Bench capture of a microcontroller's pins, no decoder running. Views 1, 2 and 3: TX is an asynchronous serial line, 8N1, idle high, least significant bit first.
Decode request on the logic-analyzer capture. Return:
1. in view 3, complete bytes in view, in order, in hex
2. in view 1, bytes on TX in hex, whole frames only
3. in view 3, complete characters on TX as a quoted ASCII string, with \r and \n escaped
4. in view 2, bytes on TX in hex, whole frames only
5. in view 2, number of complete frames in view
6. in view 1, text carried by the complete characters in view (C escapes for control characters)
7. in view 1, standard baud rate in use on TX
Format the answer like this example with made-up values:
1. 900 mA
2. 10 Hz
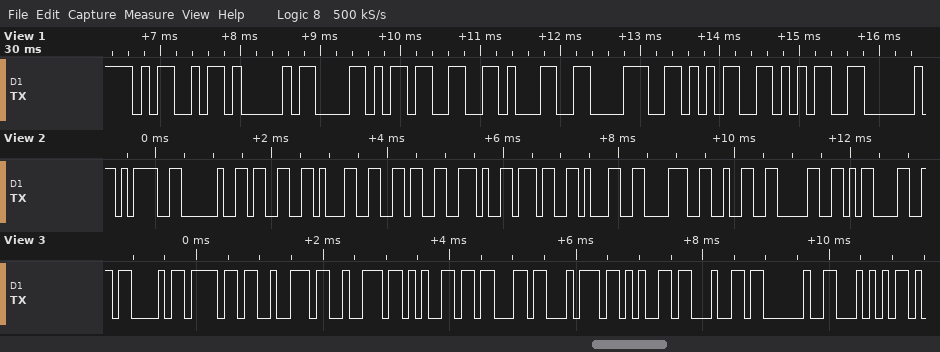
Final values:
1. 43 6F 72 72 65 63 74 65 64 20 54
2. 4D 41 58 33 31 38 35 35
3. "Corrected T"
4. 3D 20 33 31 36 2E 37 31 38 32 30 0D
5. 12
6. "MAX31855"
7. 9600 baud
